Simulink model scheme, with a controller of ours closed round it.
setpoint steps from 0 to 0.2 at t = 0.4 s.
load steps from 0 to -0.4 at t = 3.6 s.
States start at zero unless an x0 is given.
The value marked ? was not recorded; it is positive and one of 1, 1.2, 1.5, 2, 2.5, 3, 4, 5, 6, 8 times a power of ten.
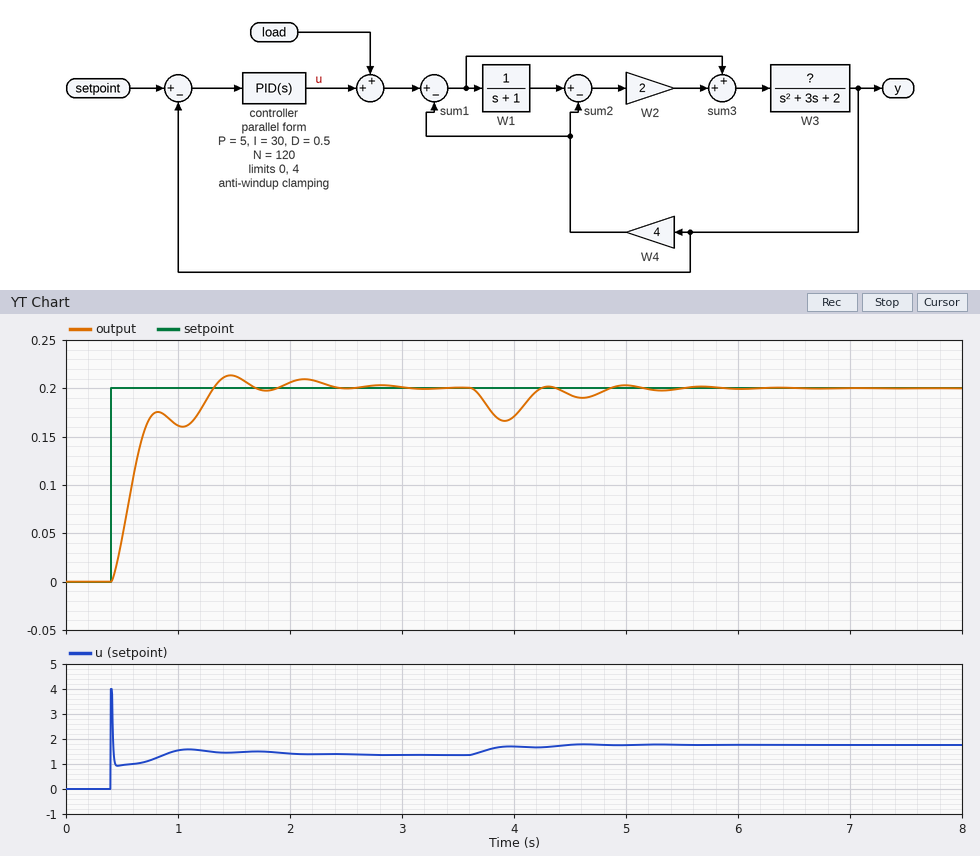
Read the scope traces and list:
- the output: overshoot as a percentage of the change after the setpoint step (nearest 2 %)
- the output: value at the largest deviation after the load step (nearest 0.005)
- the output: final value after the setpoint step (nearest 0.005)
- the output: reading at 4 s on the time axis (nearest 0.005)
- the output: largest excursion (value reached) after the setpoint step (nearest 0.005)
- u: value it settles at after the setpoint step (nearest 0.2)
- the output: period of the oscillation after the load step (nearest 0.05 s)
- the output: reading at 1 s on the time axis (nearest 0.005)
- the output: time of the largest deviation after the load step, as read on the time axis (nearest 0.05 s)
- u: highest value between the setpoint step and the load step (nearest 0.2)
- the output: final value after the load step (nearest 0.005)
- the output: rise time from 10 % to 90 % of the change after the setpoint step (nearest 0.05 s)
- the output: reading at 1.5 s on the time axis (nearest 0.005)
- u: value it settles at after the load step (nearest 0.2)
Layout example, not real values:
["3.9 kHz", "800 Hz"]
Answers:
["6 %", "0.165", "0.200", "0.170", "0.215", "1.4", "0.70 s", "0.160", "3.90 s", "4.0", "0.200", "0.75 s", "0.215", "1.8"]
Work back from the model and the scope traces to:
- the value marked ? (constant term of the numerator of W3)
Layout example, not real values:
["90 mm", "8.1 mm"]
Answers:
["5"]
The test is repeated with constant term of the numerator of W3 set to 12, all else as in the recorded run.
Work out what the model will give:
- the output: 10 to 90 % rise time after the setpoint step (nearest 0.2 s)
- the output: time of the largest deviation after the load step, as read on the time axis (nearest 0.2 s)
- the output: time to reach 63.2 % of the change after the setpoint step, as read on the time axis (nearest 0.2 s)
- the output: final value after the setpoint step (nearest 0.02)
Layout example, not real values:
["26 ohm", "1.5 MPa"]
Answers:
["0.6 s", "3.8 s", "0.6 s", "0.20"]
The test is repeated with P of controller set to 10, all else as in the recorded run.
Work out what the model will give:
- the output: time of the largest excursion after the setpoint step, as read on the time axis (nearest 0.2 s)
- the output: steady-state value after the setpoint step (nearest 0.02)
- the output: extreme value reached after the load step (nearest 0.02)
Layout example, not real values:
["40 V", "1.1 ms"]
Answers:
["1.4 s", "0.20", "0.18"]
